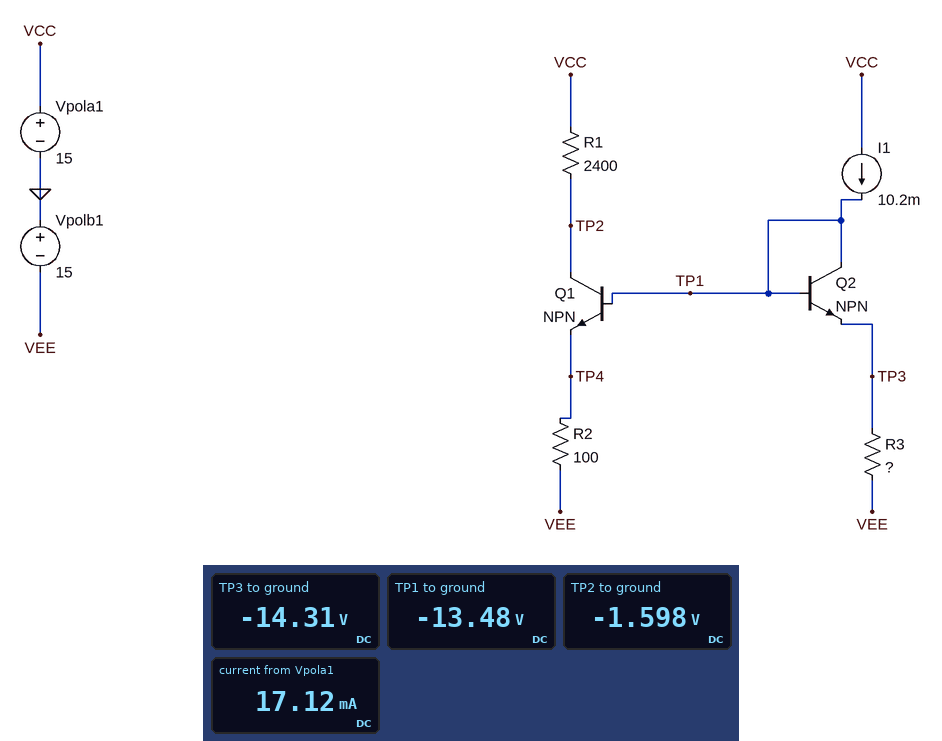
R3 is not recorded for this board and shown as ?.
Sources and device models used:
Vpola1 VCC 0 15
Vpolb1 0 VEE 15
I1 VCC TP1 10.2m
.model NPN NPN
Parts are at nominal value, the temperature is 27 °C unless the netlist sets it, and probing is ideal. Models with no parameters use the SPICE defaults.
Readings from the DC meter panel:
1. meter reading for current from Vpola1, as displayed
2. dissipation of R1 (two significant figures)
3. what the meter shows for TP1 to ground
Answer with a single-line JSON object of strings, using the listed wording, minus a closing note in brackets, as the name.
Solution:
{"meter reading for current from Vpola1, as displayed": "17.12 mA", "dissipation of R1": "110 mW", "what the meter shows for TP1 to ground": "-13.48 V"}
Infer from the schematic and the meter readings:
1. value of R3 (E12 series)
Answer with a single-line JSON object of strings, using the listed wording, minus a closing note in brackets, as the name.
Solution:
{"value of R3": "68 Ω"}
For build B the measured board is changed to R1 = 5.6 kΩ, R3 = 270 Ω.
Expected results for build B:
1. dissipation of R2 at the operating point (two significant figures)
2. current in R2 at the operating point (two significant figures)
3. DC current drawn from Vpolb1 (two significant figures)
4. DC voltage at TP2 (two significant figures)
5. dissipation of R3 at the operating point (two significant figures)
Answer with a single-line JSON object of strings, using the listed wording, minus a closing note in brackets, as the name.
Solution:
{"dissipation of R2 at the operating point": "12 mW", "current in R2 at the operating point": "11 mA", "DC current drawn from Vpolb1": "15 mA", "DC voltage at TP2": "-14 V", "dissipation of R3 at the operating point": "4.9 mW"}
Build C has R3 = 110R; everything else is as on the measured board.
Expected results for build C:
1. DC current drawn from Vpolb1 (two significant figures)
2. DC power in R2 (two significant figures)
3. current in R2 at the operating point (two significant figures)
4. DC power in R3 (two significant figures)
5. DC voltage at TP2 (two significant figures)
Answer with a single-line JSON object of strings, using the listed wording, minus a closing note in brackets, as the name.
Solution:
{"DC current drawn from Vpolb1": "21 mA", "DC power in R2": "12 mW", "current in R2 at the operating point": "11 mA", "DC power in R3": "11 mW", "DC voltage at TP2": "-11 V"}
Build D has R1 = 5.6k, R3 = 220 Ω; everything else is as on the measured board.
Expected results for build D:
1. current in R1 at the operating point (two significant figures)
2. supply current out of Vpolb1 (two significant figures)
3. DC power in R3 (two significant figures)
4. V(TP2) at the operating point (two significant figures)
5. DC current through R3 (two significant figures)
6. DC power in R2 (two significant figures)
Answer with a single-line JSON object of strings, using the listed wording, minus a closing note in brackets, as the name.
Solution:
{"current in R1 at the operating point": "5.2 mA", "supply current out of Vpolb1": "15 mA", "DC power in R3": "5.3 mW", "V(TP2) at the operating point": "-14 V", "DC current through R3": "4.9 mA", "DC power in R2": "11 mW"}
